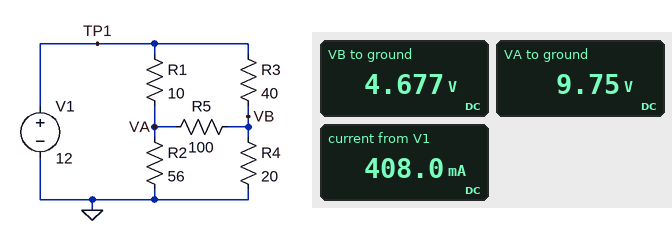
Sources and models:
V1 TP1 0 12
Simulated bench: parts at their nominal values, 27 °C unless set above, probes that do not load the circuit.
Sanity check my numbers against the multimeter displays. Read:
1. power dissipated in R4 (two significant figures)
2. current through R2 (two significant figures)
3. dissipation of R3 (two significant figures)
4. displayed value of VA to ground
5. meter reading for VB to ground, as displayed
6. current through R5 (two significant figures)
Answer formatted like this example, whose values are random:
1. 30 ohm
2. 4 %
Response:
1. 1.1 W
2. 170 mA
3. 1.3 W
4. 9.75 V
5. 4.677 V
6. 51 mA
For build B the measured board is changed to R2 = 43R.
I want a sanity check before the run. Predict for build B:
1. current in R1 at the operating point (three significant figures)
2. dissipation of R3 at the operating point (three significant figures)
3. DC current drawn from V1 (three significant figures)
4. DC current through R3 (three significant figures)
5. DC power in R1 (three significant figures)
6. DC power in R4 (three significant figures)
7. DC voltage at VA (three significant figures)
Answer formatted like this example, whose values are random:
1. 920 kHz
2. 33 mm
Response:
1. 265 mA
2. 1.36 W
3. 449 mA
4. 184 mA
5. 701 mW
6. 1.07 W
7. 9.35 V
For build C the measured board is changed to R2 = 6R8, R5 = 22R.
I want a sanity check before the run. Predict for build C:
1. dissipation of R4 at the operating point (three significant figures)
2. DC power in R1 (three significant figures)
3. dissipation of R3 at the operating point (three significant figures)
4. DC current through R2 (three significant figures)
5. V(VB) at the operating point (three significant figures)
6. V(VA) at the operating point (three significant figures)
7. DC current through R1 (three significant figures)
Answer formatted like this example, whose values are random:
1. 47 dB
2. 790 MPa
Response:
1. 920 mW
2. 5.23 W
3. 1.49 W
4. 701 mA
5. 4.29 V
6. 4.77 V
7. 723 mA
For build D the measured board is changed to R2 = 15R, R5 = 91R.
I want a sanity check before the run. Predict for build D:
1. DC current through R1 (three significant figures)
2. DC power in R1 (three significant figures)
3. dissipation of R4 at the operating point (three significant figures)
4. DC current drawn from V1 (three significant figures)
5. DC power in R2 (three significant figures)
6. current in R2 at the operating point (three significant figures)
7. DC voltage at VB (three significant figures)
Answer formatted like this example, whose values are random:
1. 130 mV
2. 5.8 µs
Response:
1. 497 mA
2. 2.47 W
3. 962 mW
4. 688 mA
5. 3.29 W
6. 468 mA
7. 4.39 V
